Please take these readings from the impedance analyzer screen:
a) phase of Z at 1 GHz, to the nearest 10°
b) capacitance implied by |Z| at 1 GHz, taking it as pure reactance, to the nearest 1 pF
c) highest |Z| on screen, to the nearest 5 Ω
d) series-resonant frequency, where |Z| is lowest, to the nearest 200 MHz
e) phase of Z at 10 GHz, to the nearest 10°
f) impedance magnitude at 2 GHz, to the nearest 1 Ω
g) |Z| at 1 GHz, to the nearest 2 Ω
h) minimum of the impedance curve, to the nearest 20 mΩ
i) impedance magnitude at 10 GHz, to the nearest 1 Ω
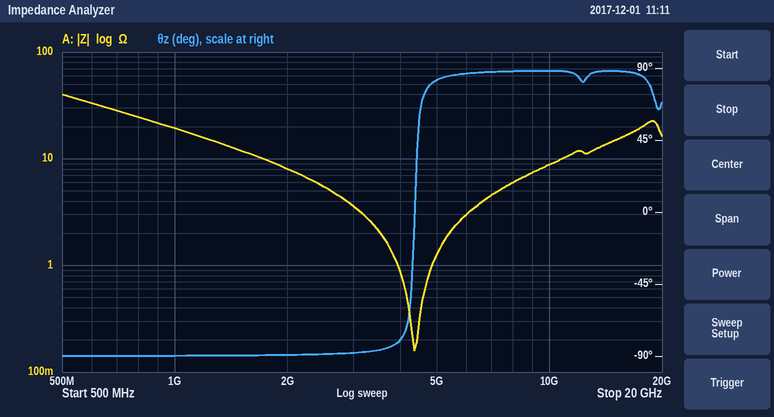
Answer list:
-90°
8 pF
40 Ω
4.4 GHz
90°
8 Ω
20 Ω
160 mΩ
9 Ω
